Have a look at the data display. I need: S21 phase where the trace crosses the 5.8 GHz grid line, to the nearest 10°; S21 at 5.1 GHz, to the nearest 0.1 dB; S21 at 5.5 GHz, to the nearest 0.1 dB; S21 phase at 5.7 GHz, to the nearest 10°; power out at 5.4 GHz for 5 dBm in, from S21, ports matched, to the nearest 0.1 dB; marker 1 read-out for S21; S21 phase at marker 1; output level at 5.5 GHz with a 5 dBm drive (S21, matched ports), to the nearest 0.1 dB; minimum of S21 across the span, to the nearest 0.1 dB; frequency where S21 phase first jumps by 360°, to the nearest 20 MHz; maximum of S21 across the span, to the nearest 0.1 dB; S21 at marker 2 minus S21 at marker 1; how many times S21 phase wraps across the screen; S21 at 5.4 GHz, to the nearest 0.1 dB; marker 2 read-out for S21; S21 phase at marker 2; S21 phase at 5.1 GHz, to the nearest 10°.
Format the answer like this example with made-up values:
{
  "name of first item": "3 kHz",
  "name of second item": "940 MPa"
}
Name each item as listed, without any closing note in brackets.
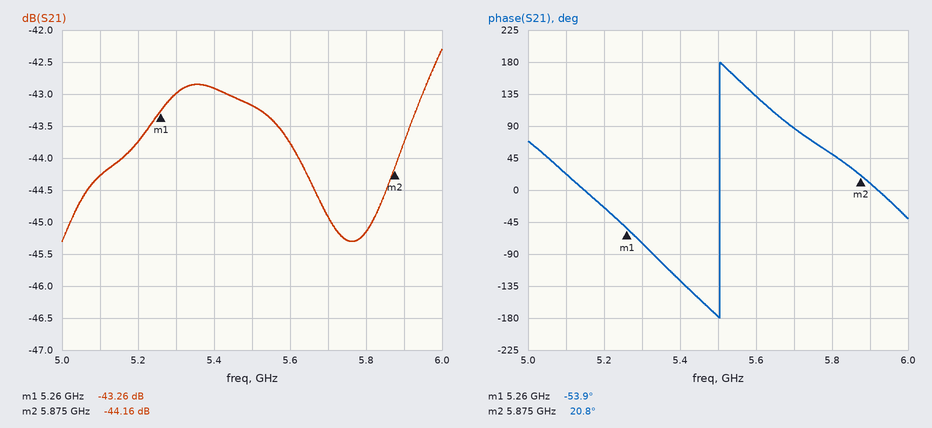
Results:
{
  "S21 phase where the trace crosses the 5.8 GHz grid line, to the nearest 10°": "50°",
  "S21 at 5.1 GHz, to the nearest 0.1 dB": "-44.3 dB",
  "S21 at 5.5 GHz, to the nearest 0.1 dB": "-43.2 dB",
  "S21 phase at 5.7 GHz, to the nearest 10°": "90°",
  "power out at 5.4 GHz for 5 dBm in, from S21, ports matched, to the nearest 0.1 dB": "-37.9 dBm",
  "marker 1 read-out for S21": "-43.26 dB",
  "S21 phase at marker 1": "-53.9°",
  "output level at 5.5 GHz with a 5 dBm drive (S21, matched ports), to the nearest 0.1 dB": "-38.2 dBm",
  "minimum of S21 across the span, to the nearest 0.1 dB": "-45.3 dB",
  "frequency where S21 phase first jumps by 360°, to the nearest 20 MHz": "5.50 GHz",
  "maximum of S21 across the span, to the nearest 0.1 dB": "-42.3 dB",
  "S21 at marker 2 minus S21 at marker 1": "-0.90 dB",
  "how many times S21 phase wraps across the screen": "1",
  "S21 at 5.4 GHz, to the nearest 0.1 dB": "-42.9 dB",
  "marker 2 read-out for S21": "-44.16 dB",
  "S21 phase at marker 2": "20.8°",
  "S21 phase at 5.1 GHz, to the nearest 10°": "20°"
}
